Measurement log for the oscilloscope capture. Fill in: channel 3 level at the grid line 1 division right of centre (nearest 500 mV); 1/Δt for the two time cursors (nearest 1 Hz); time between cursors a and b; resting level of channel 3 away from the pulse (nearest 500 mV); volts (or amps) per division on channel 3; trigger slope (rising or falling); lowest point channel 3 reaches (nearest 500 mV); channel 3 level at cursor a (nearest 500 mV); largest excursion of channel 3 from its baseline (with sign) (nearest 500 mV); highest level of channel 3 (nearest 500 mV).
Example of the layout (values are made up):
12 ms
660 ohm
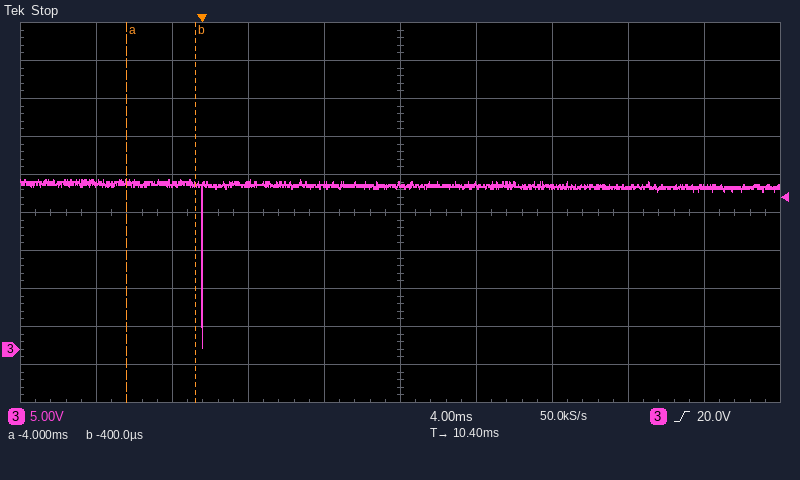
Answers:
21.5 V
278 Hz
3.6 ms
21.5 V
5 V
rising
0.0 V
22.0 V
-21.5 V
22.5 V
